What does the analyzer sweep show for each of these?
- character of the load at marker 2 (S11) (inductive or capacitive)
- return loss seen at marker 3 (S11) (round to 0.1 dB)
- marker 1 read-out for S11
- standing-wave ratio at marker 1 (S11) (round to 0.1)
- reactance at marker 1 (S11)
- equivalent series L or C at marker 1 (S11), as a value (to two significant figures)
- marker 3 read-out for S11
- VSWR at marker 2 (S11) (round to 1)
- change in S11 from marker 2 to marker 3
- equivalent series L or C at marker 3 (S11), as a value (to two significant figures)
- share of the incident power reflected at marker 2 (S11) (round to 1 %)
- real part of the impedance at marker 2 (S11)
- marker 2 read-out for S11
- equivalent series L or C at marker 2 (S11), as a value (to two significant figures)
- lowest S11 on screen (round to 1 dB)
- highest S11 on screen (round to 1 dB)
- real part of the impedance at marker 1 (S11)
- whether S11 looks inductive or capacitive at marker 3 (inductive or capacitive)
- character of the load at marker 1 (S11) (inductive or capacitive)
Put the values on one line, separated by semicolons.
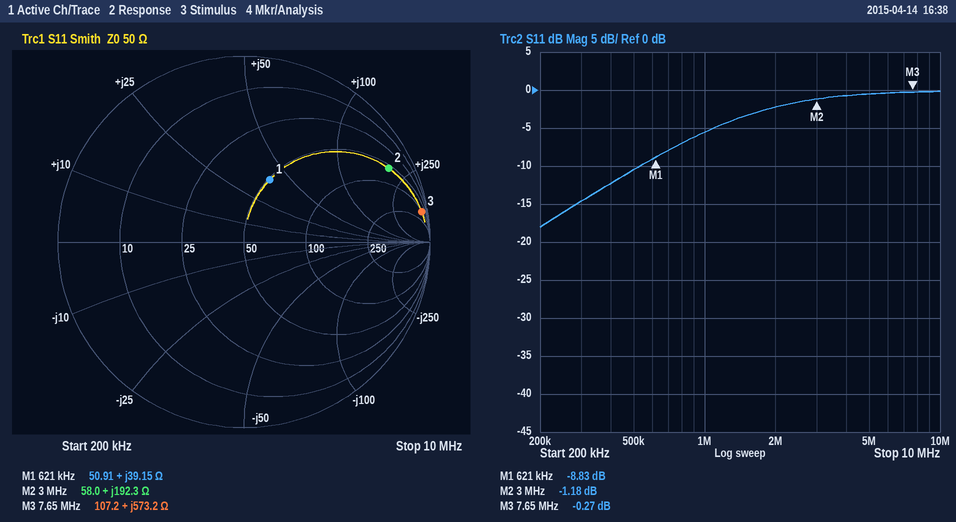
inductive; 0.3 dB; -8.83 dB; 2.1; +39.15 Ω; 10 µH; -0.27 dB; 15; 0.91 dB; 12 µH; 76 %; 58.0 Ω; -1.18 dB; 10 µH; -18 dB; 0 dB; 50.91 Ω; inductive; inductive
